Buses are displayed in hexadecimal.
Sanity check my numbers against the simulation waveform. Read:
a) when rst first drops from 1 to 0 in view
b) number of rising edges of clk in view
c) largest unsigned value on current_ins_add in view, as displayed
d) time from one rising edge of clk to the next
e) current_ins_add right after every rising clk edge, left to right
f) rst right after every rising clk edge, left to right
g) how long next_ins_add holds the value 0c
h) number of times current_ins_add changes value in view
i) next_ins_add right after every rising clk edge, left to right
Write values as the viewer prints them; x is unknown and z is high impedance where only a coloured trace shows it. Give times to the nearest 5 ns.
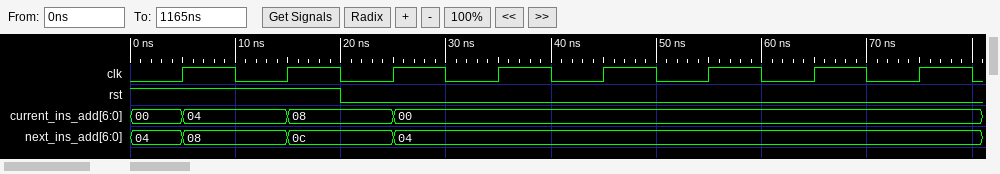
20 ns
8
08
10 ns
04, 08, 00, 00, 00, 00, 00, 00
1 1 0 0 0 0 0 0
10 ns
3
08, 0c, 04, 04, 04, 04, 04, 04
